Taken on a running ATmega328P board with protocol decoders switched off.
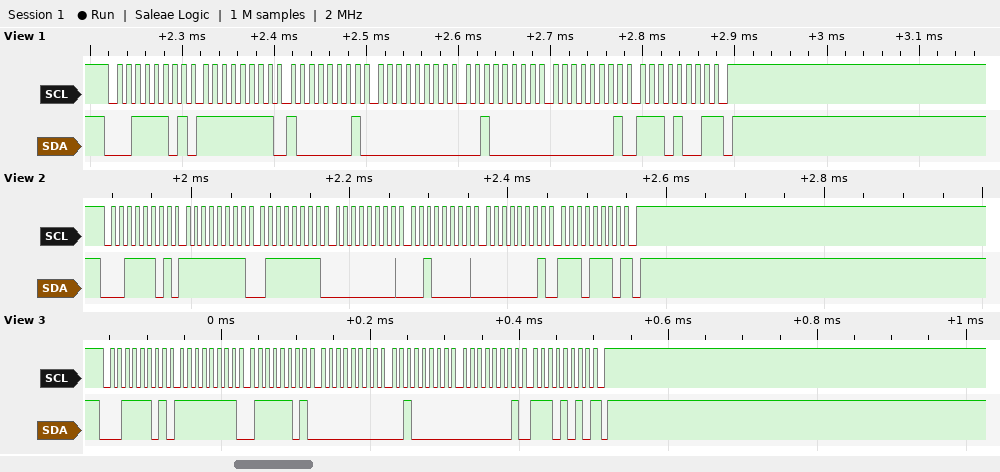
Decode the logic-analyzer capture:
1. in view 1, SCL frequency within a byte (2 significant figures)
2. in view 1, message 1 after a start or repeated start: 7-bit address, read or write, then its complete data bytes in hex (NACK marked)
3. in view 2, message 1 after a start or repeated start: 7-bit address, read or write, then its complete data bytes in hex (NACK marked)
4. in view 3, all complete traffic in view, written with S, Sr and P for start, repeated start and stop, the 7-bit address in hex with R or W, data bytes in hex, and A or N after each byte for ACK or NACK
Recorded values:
100 kHz
0x1E read: FF 81 00 20 01 E9 NACK
0x1E read: FF 7F 00 20 01 EE NACK
S 1ER A FF A 7D A 00 A 20 A 01 A EA N P
